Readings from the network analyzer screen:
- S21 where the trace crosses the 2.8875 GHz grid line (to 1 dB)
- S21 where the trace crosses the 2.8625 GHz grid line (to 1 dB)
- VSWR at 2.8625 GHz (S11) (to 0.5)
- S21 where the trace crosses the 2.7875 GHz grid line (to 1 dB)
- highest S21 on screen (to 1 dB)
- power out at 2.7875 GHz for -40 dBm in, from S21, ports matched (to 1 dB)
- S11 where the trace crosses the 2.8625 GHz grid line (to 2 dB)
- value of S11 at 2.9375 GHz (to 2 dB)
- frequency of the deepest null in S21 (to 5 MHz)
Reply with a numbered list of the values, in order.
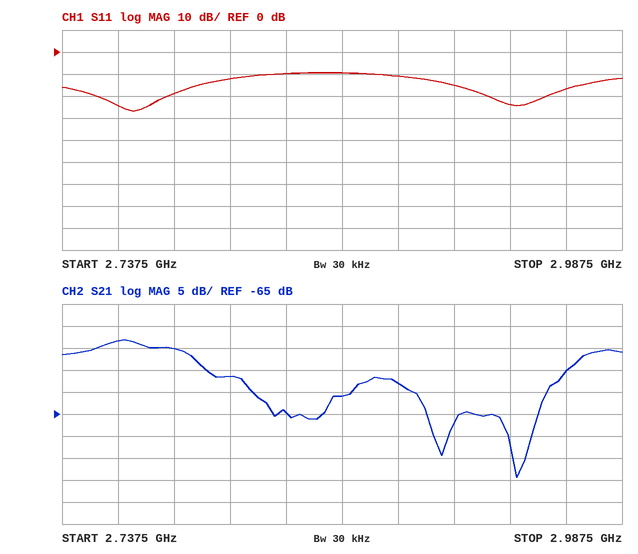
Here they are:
1. -58 dB
2. -61 dB
3. 2.0
4. -50 dB
5. -48 dB
6. -90 dBm
7. -10 dB
8. -24 dB
9. 2.940 GHz
